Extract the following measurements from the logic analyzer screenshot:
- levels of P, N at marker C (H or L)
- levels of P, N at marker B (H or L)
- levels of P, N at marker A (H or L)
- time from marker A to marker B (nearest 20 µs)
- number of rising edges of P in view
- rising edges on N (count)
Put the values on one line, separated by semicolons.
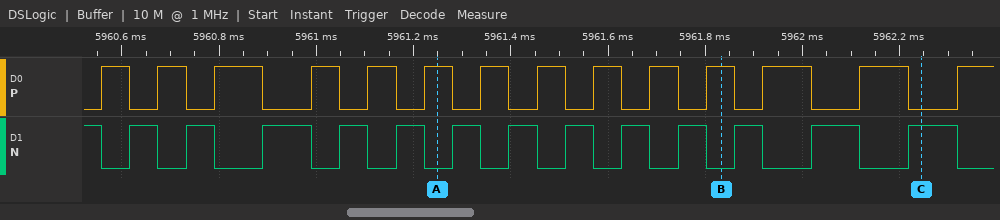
P=L, N=H; P=H, N=L; P=H, N=L; 580 µs; 14; 13
